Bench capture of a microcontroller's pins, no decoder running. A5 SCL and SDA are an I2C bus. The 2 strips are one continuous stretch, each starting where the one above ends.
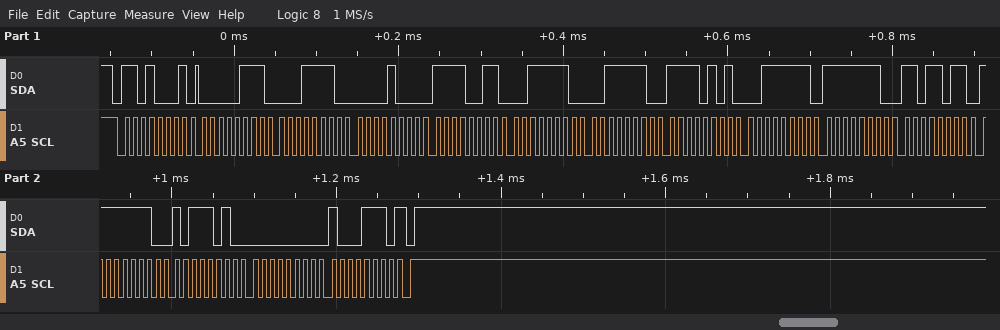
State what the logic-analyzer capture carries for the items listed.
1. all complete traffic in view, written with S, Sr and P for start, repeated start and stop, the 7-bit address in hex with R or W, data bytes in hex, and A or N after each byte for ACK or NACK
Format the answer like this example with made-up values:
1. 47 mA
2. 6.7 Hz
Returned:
1. S 68R A 07 A 1E A 08 A F3 A 3E A 3E A F5 A 3F A FE A DB A FE A BA A 00 A 8E N P
